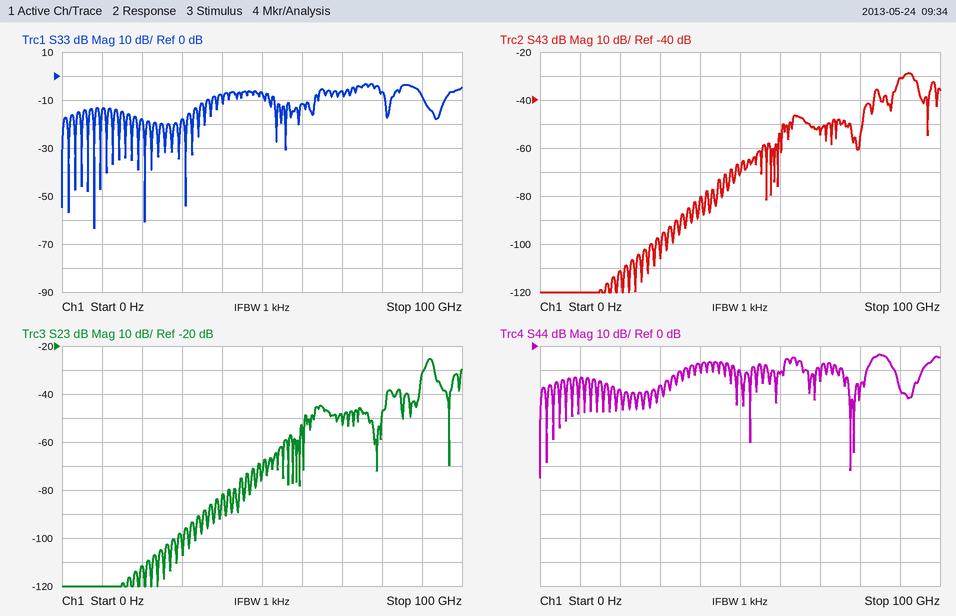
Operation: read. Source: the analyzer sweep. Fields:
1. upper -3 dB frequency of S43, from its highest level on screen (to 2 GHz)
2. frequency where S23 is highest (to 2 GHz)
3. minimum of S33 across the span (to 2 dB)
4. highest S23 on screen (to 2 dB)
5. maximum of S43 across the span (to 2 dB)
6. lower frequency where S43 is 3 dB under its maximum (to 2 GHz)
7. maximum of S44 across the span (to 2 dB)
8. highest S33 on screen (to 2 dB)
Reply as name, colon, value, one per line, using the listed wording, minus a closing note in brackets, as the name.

upper -3 dB frequency of S43, from its highest level on screen: 94 GHz
frequency where S23 is highest: 92 GHz
minimum of S33 across the span: -64 dB
highest S23 on screen: -26 dB
maximum of S43 across the span: -28 dB
lower frequency where S43 is 3 dB under its maximum: 90 GHz
maximum of S44 across the span: -4 dB
highest S33 on screen: -4 dB
